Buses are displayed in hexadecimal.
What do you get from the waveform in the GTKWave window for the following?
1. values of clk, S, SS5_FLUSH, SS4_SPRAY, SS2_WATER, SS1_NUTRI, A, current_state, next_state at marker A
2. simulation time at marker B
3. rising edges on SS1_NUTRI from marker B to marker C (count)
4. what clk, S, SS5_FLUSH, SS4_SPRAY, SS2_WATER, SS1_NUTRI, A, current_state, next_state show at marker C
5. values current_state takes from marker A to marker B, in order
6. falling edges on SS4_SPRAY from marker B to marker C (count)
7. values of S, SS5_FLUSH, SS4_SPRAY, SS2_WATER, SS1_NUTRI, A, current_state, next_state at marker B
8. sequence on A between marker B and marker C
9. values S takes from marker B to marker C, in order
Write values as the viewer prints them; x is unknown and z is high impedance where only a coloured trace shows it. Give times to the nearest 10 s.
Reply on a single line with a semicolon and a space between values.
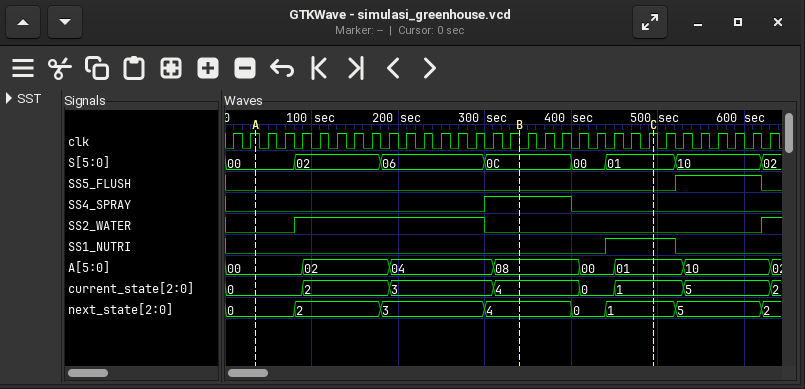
clk=1, S=00, SS5_FLUSH=0, SS4_SPRAY=0, SS2_WATER=0, SS1_NUTRI=0, A=00, current_state=0, next_state=0; 340 s; 1; clk=1, S=01, SS5_FLUSH=0, SS4_SPRAY=0, SS2_WATER=0, SS1_NUTRI=1, A=01, current_state=1, next_state=1; 0, 2, 3, 4; 1; S=0C, SS5_FLUSH=0, SS4_SPRAY=1, SS2_WATER=0, SS1_NUTRI=0, A=08, current_state=4, next_state=4; 08, 00, 01; 0C, 00, 01
